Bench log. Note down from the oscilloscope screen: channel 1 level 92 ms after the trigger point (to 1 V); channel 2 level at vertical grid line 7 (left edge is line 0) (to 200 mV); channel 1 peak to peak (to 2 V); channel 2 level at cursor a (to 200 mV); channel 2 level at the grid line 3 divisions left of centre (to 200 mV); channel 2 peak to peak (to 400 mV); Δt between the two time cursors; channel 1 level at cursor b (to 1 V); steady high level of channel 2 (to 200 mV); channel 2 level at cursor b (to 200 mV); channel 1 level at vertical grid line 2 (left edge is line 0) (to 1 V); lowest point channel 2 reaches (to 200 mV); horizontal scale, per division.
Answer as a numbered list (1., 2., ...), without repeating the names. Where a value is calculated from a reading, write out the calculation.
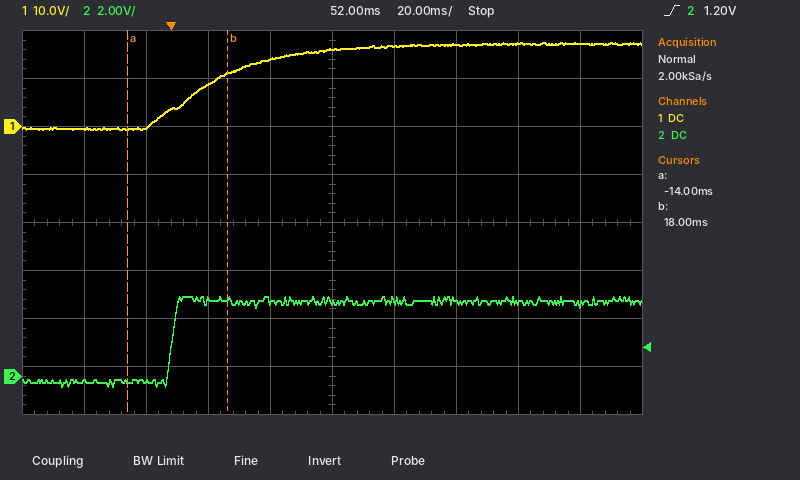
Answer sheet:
1. 17 V
2. 3.2 V
3. 18 V
4. -200 mV
5. -200 mV
6. 3.6 V
7. 18 ms − (-14 ms) = 32 ms
8. 11 V
9. 3.2 V
10. 3.2 V
11. 0 V
12. -400 mV
13. 20 ms
